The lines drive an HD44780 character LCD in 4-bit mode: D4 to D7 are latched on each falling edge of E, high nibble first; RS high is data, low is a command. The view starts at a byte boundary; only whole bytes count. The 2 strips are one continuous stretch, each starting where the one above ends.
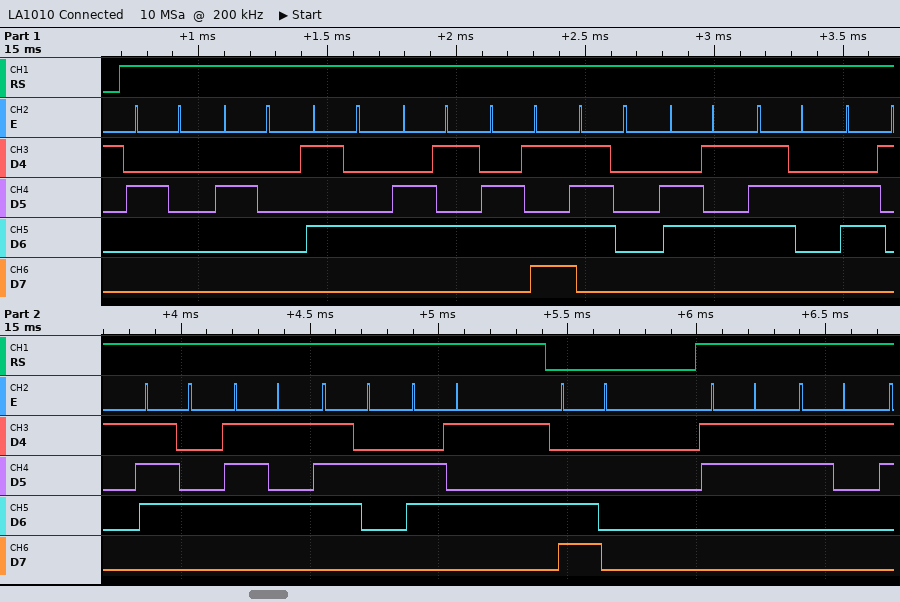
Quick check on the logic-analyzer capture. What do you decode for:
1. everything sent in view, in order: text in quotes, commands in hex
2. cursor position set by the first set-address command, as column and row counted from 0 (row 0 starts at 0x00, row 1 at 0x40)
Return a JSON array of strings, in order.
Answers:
["\"  Temperature\" 0xC0 \"31\"", "column 0, row 1"]
